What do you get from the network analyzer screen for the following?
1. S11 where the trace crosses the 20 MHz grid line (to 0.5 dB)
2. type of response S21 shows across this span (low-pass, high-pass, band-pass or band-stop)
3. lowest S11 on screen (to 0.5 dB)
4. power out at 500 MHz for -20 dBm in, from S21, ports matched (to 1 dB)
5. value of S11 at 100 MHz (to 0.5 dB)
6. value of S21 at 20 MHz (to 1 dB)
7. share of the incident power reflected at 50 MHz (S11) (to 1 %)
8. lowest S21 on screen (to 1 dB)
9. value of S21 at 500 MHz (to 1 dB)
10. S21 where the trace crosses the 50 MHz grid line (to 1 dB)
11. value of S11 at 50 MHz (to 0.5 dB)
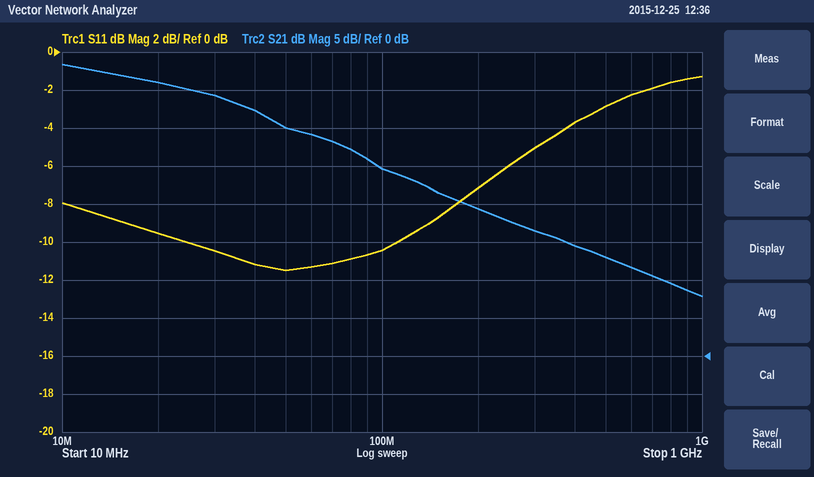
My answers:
-9.5 dB
low-pass
-11.5 dB
-7 dBm
-10.5 dB
36 dB
7 %
8 dB
13 dB
30 dB
-11.5 dB
